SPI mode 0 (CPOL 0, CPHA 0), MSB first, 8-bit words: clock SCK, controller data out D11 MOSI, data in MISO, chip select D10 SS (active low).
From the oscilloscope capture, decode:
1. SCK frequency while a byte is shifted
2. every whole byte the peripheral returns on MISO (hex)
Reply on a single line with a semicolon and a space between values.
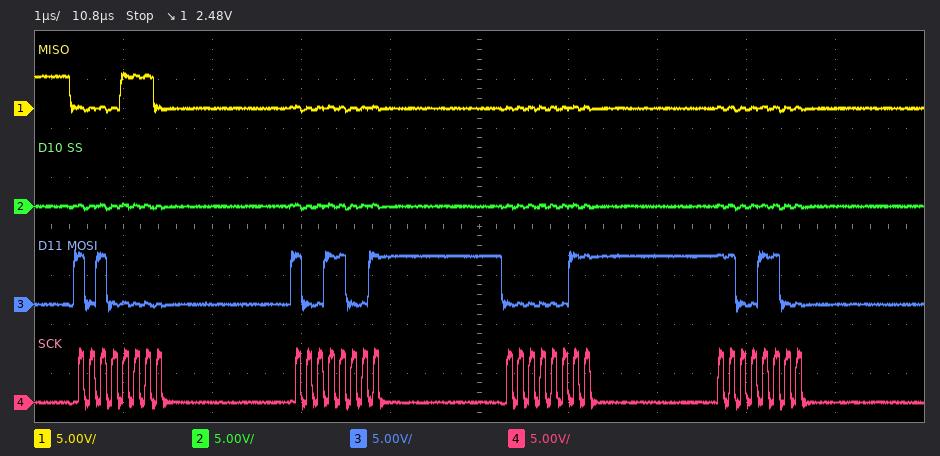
8 MHz; 0E 00 00 00
